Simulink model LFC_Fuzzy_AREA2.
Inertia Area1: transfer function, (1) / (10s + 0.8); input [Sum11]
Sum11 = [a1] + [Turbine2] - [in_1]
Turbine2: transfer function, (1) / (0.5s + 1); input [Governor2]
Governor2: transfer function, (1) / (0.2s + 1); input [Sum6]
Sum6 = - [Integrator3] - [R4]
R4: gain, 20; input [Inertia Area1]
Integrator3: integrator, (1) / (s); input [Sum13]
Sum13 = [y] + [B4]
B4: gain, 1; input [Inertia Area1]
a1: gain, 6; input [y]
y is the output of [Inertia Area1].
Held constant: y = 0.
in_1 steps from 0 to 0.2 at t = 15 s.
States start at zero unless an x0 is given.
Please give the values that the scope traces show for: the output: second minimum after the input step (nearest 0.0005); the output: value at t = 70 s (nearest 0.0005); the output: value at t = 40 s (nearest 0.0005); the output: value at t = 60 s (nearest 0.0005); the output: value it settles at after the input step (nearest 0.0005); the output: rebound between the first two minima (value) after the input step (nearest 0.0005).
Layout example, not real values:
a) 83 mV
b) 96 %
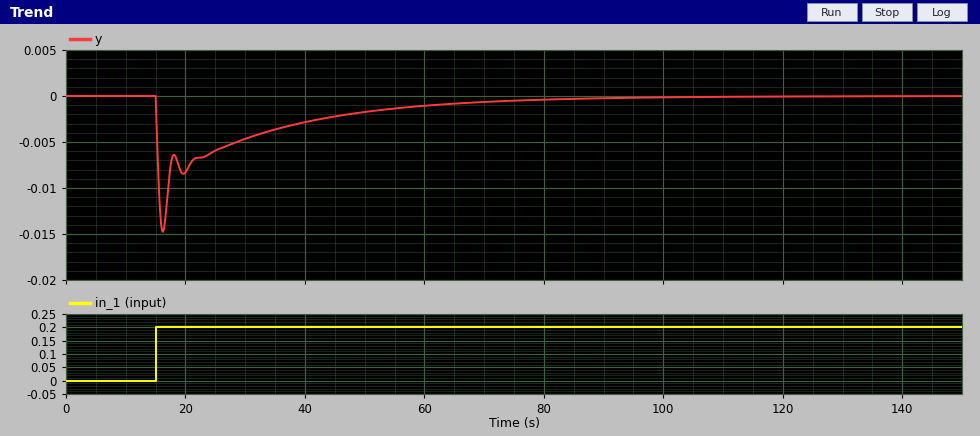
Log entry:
a) -0.0085
b) -0.0005
c) -0.0030
d) -0.0010
e) 0.0000
f) -0.0065
